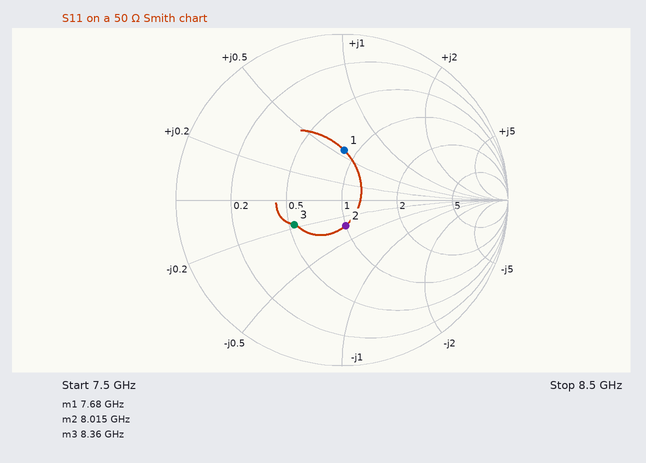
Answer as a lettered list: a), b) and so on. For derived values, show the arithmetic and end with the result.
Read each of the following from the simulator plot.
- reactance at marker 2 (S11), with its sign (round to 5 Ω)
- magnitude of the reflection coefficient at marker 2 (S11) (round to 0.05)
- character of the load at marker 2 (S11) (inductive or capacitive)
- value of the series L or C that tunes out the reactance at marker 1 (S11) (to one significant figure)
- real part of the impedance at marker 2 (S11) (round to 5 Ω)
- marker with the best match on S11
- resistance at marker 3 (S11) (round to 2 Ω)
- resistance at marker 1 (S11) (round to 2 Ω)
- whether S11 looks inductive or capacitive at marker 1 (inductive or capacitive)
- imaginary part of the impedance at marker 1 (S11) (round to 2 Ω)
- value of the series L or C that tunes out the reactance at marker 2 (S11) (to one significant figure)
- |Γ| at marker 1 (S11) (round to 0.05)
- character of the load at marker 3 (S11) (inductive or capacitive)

a) -15 Ω
b) 0.15
c) capacitive
d) C = 1/(2π × 7.68 GHz × 28 Ω) ≈ 740 fF, so 700 fF to one significant figure
e) 50 Ω
f) marker 2
g) 26 Ω
h) 42 Ω
i) inductive
j) +28 Ω
k) L = 15 Ω/(2π × 8.015 GHz) ≈ 298 pH, so 300 pH to one significant figure
l) 0.30
m) capacitive
